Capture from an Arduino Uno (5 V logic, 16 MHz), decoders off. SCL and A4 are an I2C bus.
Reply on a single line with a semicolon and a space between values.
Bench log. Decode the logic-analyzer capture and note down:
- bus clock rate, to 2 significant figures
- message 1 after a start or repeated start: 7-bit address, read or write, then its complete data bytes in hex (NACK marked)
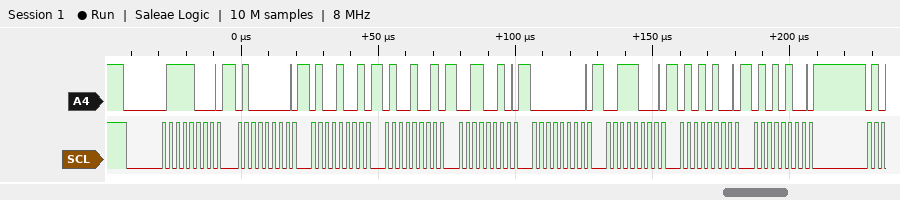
400 kHz; 0x3C write: 40 49 49 32 00 38 54 54
